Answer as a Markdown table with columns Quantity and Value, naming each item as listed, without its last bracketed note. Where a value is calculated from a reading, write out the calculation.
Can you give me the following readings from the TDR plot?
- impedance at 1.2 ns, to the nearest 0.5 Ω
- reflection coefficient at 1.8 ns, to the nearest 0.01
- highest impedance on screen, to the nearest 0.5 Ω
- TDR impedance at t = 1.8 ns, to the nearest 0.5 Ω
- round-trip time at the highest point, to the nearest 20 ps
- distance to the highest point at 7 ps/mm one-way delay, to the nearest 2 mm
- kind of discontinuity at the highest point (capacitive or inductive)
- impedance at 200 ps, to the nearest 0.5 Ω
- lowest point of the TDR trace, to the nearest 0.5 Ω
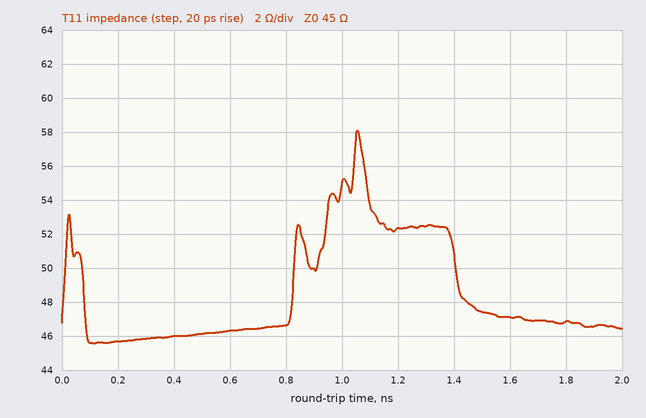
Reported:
| Quantity | Value |
|---|---|
| impedance at 1.2 ns, to the nearest 0.5 Ω | 52.5 Ω |
| reflection coefficient at 1.8 ns, to the nearest 0.01 | (47 − 45)/(47 + 45) ≈ +0.02 |
| highest impedance on screen, to the nearest 0.5 Ω | 58.0 Ω |
| TDR impedance at t = 1.8 ns, to the nearest 0.5 Ω | 47.0 Ω |
| round-trip time at the highest point, to the nearest 20 ps | 1.06 ns |
| distance to the highest point at 7 ps/mm one-way delay, to the nearest 2 mm | 1.06 ns / 2 / 7 ps/mm ≈ 76 mm |
| kind of discontinuity at the highest point | inductive |
| impedance at 200 ps, to the nearest 0.5 Ω | 45.5 Ω |
| lowest point of the TDR trace, to the nearest 0.5 Ω | 45.5 Ω |
